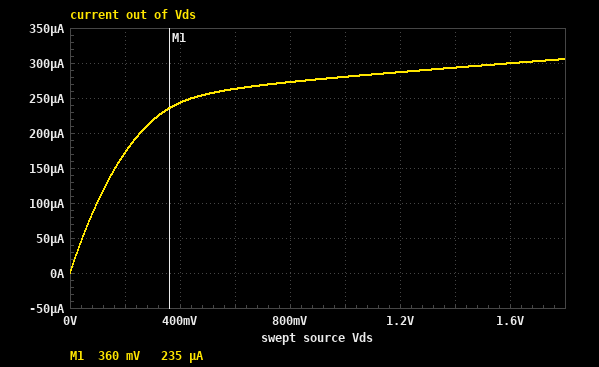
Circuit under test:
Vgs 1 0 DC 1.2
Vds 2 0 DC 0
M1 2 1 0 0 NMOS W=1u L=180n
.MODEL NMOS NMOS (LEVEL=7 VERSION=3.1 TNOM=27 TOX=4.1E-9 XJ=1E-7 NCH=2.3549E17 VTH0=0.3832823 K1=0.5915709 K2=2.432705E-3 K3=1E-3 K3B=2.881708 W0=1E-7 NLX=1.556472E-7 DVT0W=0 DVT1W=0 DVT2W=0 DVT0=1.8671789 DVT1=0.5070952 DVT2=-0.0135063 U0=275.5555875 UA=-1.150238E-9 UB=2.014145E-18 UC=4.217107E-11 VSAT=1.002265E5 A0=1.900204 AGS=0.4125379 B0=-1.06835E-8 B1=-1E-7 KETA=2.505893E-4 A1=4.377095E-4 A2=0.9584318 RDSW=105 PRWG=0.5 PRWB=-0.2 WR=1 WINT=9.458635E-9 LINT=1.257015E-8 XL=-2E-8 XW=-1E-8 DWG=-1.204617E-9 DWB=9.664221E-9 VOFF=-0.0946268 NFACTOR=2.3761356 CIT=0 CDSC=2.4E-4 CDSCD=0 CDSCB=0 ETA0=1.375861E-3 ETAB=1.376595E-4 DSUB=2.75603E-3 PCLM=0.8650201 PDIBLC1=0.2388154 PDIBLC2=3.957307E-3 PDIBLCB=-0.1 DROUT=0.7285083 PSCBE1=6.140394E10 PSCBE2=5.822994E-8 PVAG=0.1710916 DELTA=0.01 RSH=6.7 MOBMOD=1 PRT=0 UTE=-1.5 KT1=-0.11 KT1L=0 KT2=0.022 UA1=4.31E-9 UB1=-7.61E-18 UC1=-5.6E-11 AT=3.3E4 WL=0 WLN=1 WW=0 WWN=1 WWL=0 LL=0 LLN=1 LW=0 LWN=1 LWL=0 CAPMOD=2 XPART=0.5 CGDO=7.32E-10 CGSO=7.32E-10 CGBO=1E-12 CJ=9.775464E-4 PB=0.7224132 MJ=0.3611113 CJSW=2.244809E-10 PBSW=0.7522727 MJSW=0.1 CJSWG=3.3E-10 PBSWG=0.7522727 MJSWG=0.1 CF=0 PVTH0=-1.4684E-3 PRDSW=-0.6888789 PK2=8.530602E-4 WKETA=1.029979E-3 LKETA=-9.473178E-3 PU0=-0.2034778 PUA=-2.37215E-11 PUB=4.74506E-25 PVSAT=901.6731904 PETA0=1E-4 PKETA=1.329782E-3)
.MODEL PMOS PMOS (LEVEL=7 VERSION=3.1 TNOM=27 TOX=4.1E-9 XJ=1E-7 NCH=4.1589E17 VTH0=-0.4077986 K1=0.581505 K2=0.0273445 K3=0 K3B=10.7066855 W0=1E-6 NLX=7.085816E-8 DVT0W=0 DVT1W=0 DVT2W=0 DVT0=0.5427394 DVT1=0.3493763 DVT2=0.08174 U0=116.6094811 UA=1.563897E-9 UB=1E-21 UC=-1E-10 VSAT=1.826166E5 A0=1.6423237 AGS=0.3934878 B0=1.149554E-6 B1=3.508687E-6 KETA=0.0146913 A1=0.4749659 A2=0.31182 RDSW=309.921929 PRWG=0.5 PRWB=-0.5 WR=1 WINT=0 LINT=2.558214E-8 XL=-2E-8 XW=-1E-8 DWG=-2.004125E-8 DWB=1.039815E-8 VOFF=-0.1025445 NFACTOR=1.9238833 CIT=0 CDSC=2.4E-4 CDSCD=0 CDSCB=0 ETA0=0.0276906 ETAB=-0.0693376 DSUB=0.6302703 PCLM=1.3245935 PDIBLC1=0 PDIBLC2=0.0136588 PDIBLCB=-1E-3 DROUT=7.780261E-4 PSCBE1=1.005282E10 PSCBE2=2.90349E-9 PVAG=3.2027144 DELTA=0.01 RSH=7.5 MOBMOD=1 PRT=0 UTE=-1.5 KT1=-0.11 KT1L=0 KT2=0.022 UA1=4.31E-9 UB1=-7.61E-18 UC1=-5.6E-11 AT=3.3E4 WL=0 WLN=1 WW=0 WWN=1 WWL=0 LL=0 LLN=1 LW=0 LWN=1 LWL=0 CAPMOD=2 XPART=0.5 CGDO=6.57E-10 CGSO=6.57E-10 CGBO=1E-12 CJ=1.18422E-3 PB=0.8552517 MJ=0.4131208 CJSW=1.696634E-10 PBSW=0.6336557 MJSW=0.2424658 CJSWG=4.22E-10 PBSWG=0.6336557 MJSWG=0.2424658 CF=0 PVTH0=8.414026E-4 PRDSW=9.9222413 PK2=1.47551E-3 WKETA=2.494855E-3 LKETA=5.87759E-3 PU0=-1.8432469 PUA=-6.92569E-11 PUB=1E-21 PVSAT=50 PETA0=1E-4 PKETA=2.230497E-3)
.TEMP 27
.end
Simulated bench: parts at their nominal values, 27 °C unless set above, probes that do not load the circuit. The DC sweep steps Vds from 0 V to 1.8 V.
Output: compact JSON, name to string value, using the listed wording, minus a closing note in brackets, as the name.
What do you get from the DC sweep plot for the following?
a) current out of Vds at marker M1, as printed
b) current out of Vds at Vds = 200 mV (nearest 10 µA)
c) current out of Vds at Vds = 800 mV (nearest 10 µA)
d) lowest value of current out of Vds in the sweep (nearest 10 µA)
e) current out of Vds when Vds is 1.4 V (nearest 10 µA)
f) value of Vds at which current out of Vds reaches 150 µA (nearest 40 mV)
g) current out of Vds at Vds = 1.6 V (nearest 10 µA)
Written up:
{"current out of Vds at marker M1, as printed": "235 µA", "current out of Vds at Vds = 200 mV": "170 µA", "current out of Vds at Vds = 800 mV": "270 µA", "lowest value of current out of Vds in the sweep": "0 A", "current out of Vds when Vds is 1.4 V": "290 µA", "value of Vds at which current out of Vds reaches 150 µA": "160 mV", "current out of Vds at Vds = 1.6 V": "300 µA"}
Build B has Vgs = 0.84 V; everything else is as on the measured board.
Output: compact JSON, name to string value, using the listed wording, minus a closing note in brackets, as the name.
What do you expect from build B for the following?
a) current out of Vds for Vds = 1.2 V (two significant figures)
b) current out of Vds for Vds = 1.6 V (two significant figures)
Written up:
{"current out of Vds for Vds = 1.2 V": "110 µA", "current out of Vds for Vds = 1.6 V": "120 µA"}
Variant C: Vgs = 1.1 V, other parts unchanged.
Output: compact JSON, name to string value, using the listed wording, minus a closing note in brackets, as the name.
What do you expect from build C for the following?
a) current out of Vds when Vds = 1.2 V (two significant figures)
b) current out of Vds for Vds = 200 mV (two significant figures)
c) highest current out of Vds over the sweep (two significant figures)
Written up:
{"current out of Vds when Vds = 1.2 V": "240 µA", "current out of Vds for Vds = 200 mV": "150 µA", "highest current out of Vds over the sweep": "250 µA"}
